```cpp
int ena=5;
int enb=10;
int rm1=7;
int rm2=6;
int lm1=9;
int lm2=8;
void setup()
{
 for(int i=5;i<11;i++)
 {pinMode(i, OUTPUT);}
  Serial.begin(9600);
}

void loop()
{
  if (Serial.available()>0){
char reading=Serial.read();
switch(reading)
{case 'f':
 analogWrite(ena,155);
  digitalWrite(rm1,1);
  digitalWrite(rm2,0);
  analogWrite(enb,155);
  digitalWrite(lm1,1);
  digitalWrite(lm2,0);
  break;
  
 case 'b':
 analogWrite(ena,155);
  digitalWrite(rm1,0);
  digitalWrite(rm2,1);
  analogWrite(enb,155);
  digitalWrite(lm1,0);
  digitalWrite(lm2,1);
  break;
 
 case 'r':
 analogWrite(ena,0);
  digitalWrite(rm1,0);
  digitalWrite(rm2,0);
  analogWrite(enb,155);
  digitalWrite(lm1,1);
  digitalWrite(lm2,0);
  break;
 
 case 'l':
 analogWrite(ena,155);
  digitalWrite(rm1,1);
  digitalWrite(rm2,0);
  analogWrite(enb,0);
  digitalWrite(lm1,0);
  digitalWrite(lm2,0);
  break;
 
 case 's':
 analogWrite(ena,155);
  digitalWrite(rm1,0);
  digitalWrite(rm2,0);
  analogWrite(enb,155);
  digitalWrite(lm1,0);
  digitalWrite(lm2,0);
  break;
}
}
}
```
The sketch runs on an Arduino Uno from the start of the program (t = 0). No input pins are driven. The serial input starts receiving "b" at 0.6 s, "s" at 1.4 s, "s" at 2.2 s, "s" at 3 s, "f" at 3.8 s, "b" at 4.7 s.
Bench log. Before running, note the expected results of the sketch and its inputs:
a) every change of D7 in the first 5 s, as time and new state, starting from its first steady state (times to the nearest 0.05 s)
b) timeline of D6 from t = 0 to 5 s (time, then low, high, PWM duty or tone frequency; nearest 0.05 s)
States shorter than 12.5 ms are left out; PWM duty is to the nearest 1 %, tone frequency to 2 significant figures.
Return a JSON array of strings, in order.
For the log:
["0 s low; 3.8 s high; 4.7 s low", "0 s low; 0.6 s high; 1.4 s low; 4.7 s high"]
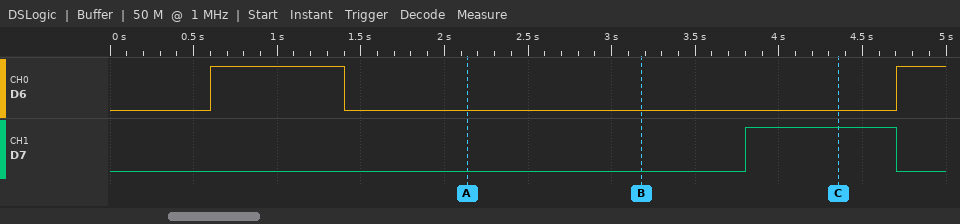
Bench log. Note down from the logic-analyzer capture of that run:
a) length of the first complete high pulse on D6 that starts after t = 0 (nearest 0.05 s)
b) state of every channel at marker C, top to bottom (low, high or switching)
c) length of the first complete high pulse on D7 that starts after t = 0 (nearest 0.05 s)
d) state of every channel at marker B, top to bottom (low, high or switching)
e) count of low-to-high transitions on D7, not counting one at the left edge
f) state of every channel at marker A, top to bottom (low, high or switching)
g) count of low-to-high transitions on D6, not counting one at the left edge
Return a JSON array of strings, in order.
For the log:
["0.80 s", "D6 low, D7 high", "0.90 s", "D6 low, D7 low", "1", "D6 low, D7 low", "2"]
